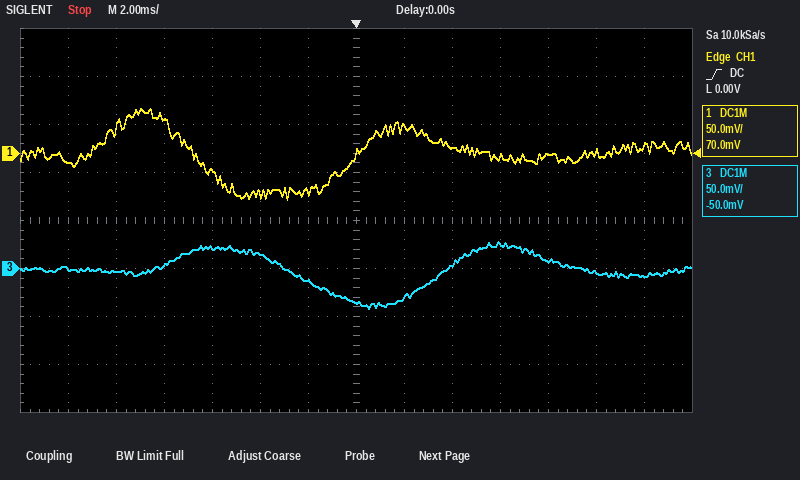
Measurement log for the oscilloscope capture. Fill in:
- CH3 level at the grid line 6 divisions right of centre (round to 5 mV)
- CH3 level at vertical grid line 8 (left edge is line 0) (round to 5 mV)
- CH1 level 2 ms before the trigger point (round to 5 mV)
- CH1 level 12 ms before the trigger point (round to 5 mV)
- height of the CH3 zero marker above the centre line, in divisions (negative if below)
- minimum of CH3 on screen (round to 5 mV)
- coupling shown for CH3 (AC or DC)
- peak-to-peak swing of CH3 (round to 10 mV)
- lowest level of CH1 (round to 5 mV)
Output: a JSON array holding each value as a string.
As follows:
["-10 mV", "-30 mV", "-40 mV", "-10 mV", "-1.0 div", "-40 mV", "DC", "70 mV", "-50 mV"]
